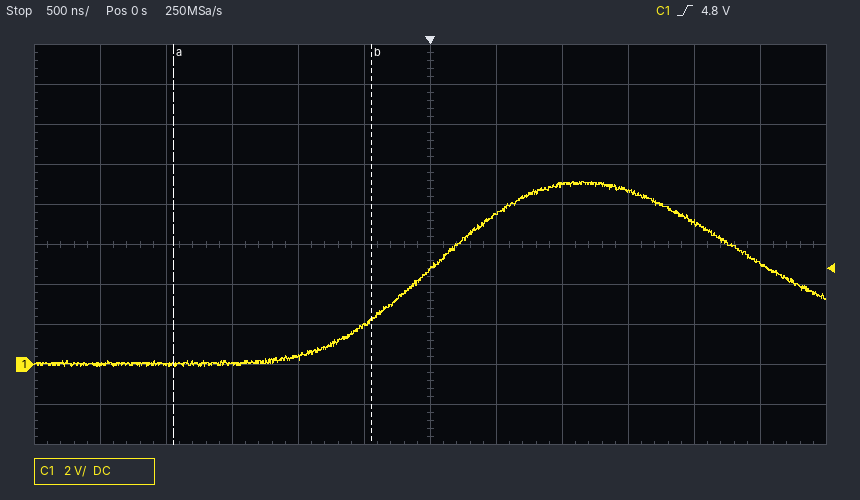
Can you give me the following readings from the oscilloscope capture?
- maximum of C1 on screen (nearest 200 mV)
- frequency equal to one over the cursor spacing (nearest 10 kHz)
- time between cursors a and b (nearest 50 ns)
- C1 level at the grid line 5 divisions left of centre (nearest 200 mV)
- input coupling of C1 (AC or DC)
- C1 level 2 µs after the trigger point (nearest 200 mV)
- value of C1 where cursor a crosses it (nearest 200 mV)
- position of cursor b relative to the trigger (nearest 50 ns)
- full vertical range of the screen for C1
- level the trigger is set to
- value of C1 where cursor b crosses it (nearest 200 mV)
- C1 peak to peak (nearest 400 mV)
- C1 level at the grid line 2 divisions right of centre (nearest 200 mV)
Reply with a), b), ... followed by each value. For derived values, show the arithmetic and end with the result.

a) 9.2 V
b) 1 / 1.50 µs ≈ 670 kHz
c) 1.50 µs
d) 0.0 V
e) DC
f) 7.0 V
g) 0.0 V
h) -450 ns
i) 20 V
j) 4.8 V
k) 2.2 V
l) 9.2 V
m) 9.0 V
